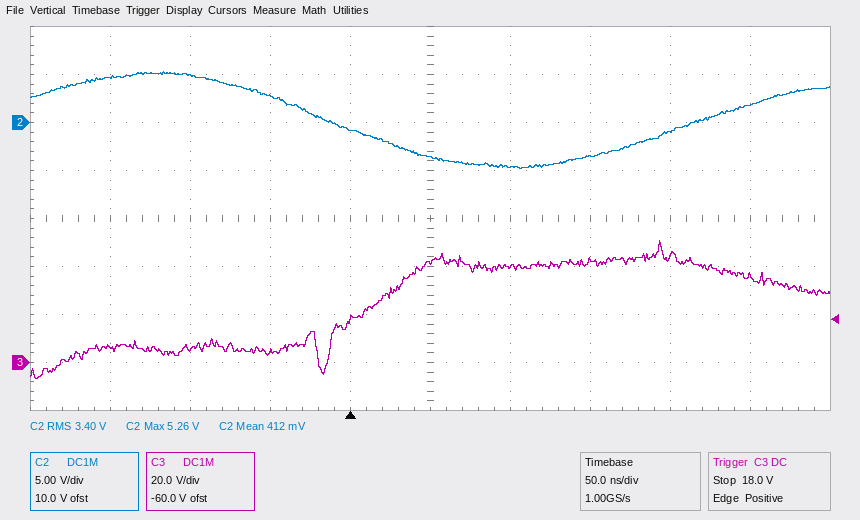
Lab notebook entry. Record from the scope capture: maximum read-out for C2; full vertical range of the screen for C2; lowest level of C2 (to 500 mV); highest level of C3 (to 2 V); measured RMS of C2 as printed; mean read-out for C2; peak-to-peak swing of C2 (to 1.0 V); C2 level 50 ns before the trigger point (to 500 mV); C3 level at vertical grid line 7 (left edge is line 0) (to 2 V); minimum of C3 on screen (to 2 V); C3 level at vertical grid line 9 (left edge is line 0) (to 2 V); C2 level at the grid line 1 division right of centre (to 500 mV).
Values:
5.26 V
40 V
-5.0 V
50 V
3.40 V
412 mV
10.0 V
2.5 V
42 V
-6 V
36 V
-4.5 V
